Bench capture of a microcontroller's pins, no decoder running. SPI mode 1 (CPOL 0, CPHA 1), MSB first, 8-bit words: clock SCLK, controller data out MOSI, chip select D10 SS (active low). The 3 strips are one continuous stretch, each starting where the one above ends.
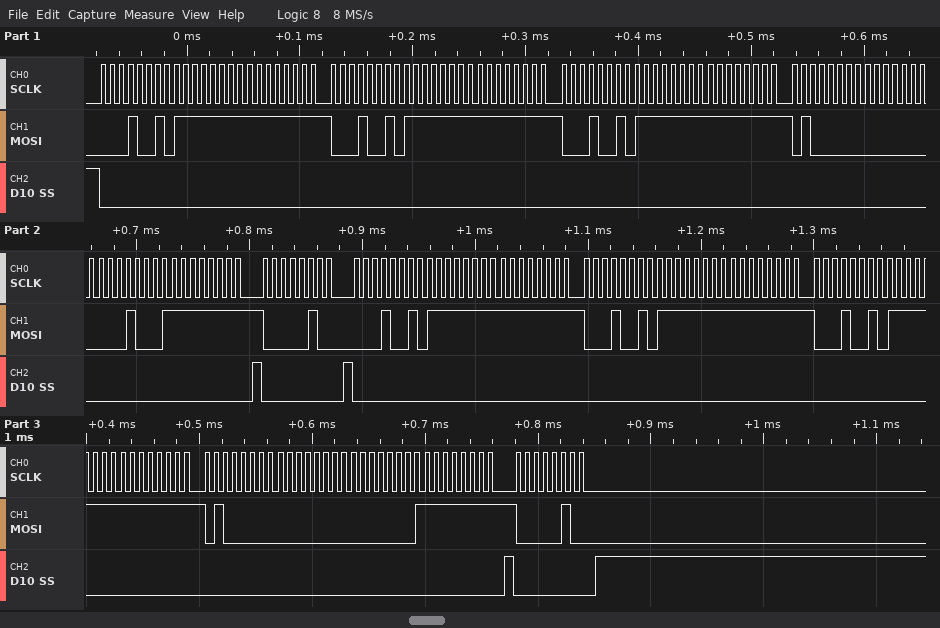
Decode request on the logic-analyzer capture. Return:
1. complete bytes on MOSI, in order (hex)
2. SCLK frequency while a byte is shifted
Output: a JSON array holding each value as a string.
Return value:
["12 FF FF 12 FF FF 12 FF FF 40 00 11 FF 04 12 FF FF 12 FF FF 12 FF FF 40 00 01 FF 04", "125 kHz"]
